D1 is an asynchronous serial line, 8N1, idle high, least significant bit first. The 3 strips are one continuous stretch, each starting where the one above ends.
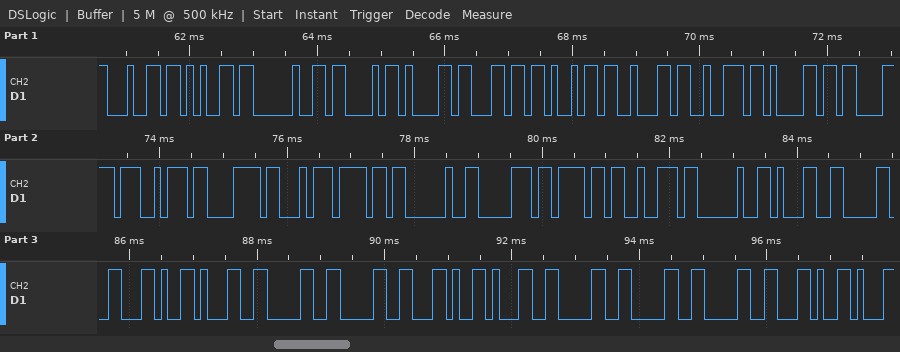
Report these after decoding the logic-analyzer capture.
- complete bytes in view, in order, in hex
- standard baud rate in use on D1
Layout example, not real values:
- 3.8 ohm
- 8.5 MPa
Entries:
- 64 65 20 43 61 6C 69 62 72 61 C3 A7 C3 A3 6F 20 70 6F 72 20 31 30 2C 31 30 30 2C 31 30 30 30 2C
- 9600 baud
